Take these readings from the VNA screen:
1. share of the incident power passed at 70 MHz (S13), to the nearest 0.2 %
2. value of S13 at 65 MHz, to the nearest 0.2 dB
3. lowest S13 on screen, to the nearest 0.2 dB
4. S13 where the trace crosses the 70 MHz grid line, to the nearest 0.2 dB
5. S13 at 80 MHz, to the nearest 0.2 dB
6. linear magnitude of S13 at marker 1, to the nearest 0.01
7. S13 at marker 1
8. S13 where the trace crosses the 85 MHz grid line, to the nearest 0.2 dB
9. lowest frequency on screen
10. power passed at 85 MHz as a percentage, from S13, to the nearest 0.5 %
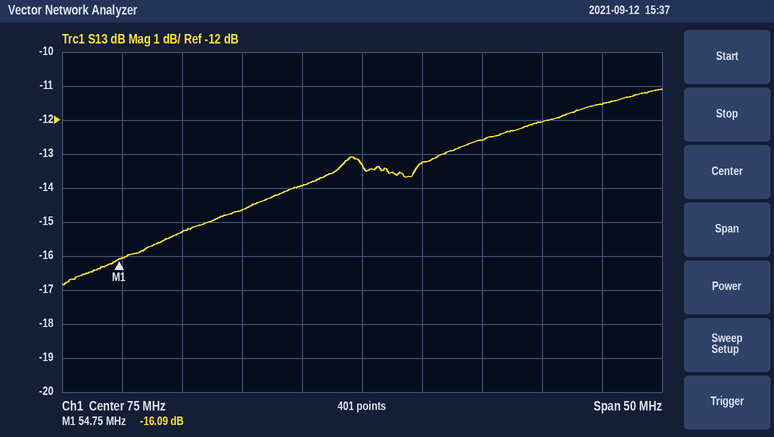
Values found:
4.0 %
-14.6 dB
-16.8 dB
-14.0 dB
-13.2 dB
0.16
-16.09 dB
-12.6 dB
50 MHz
5.5 %
